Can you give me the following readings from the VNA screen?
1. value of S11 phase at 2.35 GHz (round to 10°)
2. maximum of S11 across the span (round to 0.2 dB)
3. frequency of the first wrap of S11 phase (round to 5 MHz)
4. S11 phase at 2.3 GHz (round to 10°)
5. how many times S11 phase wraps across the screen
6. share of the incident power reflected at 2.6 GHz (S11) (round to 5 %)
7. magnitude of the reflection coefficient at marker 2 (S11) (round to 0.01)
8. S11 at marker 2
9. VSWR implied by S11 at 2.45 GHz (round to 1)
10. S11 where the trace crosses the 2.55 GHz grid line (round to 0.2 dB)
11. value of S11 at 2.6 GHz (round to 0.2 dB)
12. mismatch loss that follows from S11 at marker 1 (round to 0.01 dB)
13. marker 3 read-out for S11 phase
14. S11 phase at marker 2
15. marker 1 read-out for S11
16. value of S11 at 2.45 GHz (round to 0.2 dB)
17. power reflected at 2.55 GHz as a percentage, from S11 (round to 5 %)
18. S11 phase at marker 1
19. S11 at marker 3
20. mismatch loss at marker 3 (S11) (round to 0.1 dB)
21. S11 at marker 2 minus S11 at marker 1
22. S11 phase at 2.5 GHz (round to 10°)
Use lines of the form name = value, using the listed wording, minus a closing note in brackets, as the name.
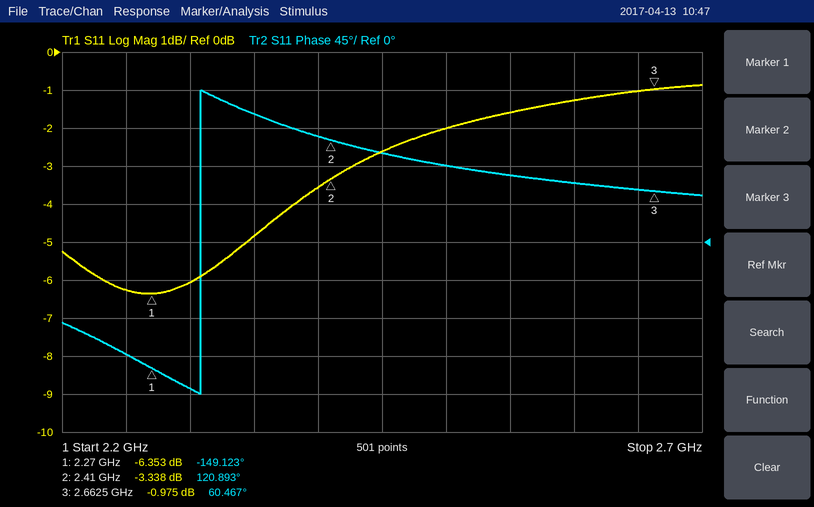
value of S11 phase at 2.35 GHz = 150°
maximum of S11 across the span = -0.8 dB
frequency of the first wrap of S11 phase = 2.310 GHz
S11 phase at 2.3 GHz = -170°
how many times S11 phase wraps across the screen = 1
share of the incident power reflected at 2.6 GHz (S11) = 75 %
magnitude of the reflection coefficient at marker 2 (S11) = 0.68
S11 at marker 2 = -3.338 dB
VSWR implied by S11 at 2.45 GHz = 7
S11 where the trace crosses the 2.55 GHz grid line = -1.6 dB
value of S11 at 2.6 GHz = -1.2 dB
mismatch loss that follows from S11 at marker 1 = 1.14 dB
marker 3 read-out for S11 phase = 60.467°
S11 phase at marker 2 = 120.893°
marker 1 read-out for S11 = -6.353 dB
value of S11 at 2.45 GHz = -2.6 dB
power reflected at 2.55 GHz as a percentage, from S11 = 70 %
S11 phase at marker 1 = -149.123°
S11 at marker 3 = -0.975 dB
mismatch loss at marker 3 (S11) = 7.0 dB
S11 at marker 2 minus S11 at marker 1 = 3.015 dB
S11 phase at 2.5 GHz = 90°
